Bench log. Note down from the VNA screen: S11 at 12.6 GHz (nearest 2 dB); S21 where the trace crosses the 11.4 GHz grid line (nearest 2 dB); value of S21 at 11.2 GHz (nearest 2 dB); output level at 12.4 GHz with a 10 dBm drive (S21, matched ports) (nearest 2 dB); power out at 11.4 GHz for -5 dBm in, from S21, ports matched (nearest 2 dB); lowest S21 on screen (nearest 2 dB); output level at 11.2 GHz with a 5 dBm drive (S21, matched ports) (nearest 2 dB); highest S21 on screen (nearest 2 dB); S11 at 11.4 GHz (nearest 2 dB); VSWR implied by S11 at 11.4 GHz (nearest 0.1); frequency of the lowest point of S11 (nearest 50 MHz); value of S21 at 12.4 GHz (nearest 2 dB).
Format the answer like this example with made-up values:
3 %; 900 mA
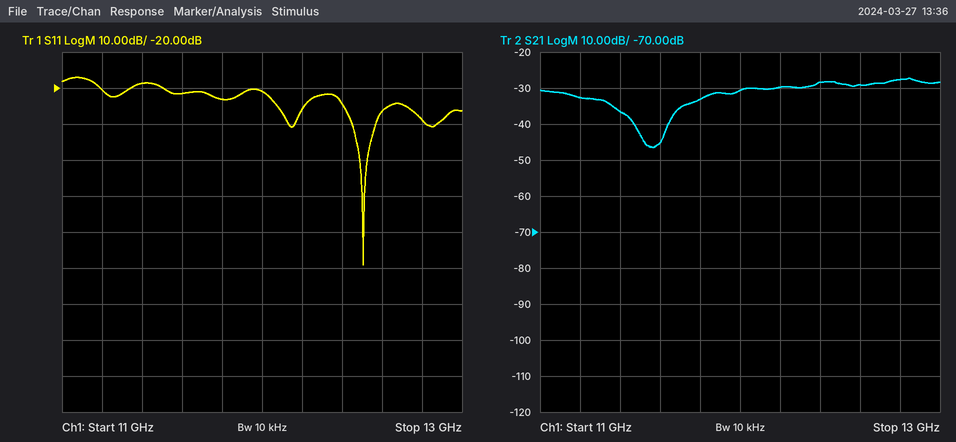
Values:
-26 dB; -36 dB; -32 dB; -18 dBm; -42 dBm; -46 dB; -28 dBm; -28 dB; -18 dB; 1.3; 12.50 GHz; -28 dB
